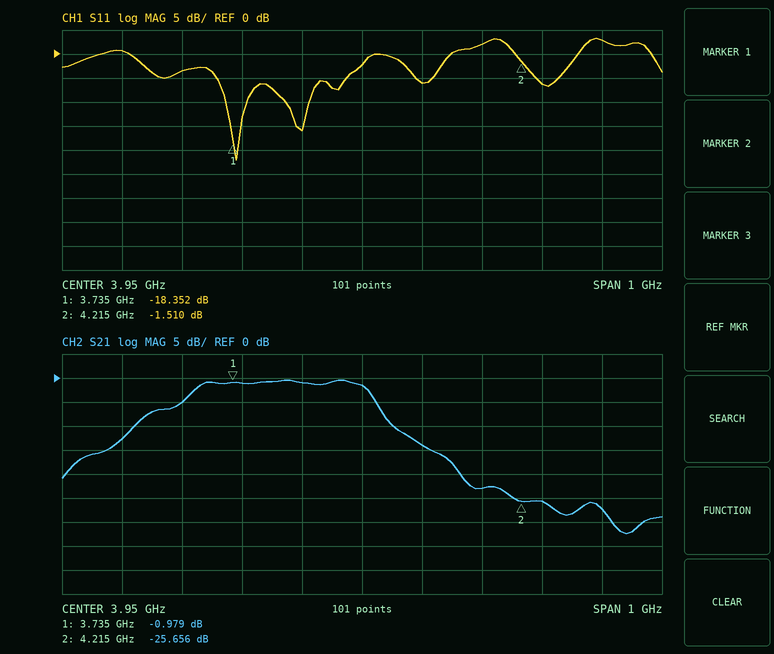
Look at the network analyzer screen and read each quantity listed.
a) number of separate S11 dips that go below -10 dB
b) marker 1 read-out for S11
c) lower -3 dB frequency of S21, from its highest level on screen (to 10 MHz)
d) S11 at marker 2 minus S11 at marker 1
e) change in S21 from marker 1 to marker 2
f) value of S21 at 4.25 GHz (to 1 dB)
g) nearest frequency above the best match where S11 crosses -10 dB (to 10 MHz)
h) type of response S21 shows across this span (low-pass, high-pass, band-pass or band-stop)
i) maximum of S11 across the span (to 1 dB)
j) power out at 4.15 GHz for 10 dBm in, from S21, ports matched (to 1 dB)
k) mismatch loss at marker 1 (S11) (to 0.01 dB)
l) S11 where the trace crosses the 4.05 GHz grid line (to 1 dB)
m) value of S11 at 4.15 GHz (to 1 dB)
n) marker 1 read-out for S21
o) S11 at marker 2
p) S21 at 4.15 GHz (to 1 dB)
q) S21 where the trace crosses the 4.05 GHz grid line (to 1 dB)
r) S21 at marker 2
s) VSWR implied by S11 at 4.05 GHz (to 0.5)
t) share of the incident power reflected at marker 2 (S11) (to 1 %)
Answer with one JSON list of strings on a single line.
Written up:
["2", "-18.352 dB", "3.66 GHz", "16.842 dB", "-24.677 dB", "-26 dB", "3.76 GHz", "band-pass", "3 dB", "-13 dBm", "0.06 dB", "-6 dB", "2 dB", "-0.979 dB", "-1.510 dB", "-23 dB", "-14 dB", "-25.656 dB", "3.0", "71 %"]
